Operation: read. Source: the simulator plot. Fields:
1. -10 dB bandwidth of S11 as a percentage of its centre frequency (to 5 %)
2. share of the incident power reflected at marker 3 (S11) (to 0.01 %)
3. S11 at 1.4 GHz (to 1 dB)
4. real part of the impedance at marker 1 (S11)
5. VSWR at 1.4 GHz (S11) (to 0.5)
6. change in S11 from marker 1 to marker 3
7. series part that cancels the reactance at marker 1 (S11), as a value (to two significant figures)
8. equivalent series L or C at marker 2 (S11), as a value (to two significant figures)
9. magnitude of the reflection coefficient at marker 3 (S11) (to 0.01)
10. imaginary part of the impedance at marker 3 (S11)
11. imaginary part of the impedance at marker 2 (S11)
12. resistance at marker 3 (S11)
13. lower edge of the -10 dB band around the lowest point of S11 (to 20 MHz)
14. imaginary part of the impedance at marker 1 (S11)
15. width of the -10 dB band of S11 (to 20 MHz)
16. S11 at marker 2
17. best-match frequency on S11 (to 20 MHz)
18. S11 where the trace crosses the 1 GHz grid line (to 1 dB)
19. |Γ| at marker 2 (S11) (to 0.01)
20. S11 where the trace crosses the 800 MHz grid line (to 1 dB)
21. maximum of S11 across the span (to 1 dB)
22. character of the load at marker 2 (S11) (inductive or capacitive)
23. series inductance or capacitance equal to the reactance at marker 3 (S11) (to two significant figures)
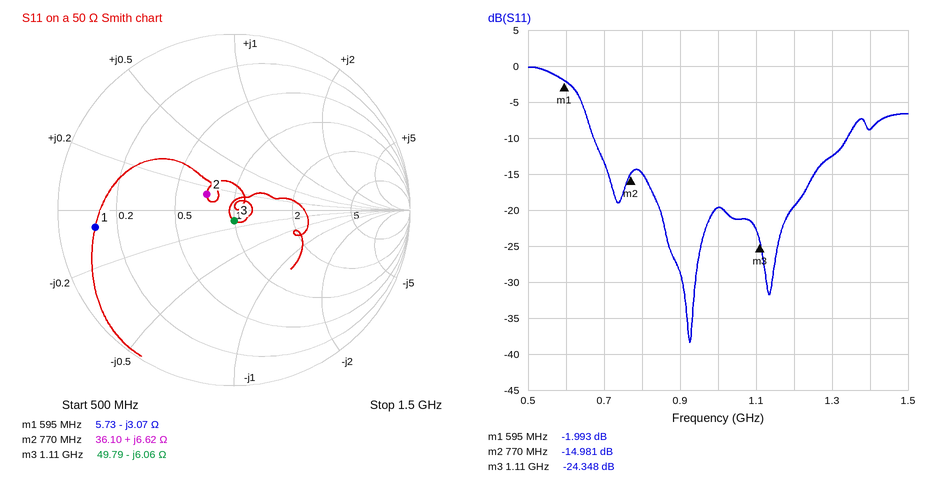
65 %
0.37 %
-9 dB
5.73 Ω
2.0
-22.355 dB
820 pH
1.4 nH
0.06
-6.06 Ω
+6.62 Ω
49.79 Ω
680 MHz
-3.07 Ω
660 MHz
-14.981 dB
920 MHz
-20 dB
0.18
-15 dB
0 dB
inductive
24 pF
